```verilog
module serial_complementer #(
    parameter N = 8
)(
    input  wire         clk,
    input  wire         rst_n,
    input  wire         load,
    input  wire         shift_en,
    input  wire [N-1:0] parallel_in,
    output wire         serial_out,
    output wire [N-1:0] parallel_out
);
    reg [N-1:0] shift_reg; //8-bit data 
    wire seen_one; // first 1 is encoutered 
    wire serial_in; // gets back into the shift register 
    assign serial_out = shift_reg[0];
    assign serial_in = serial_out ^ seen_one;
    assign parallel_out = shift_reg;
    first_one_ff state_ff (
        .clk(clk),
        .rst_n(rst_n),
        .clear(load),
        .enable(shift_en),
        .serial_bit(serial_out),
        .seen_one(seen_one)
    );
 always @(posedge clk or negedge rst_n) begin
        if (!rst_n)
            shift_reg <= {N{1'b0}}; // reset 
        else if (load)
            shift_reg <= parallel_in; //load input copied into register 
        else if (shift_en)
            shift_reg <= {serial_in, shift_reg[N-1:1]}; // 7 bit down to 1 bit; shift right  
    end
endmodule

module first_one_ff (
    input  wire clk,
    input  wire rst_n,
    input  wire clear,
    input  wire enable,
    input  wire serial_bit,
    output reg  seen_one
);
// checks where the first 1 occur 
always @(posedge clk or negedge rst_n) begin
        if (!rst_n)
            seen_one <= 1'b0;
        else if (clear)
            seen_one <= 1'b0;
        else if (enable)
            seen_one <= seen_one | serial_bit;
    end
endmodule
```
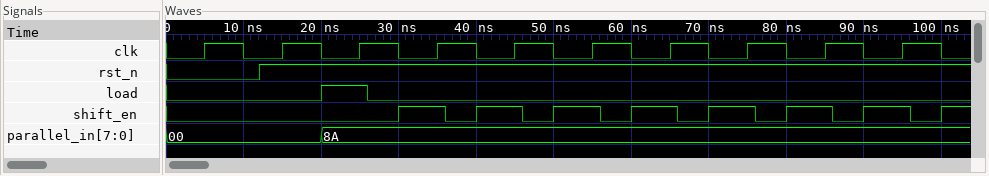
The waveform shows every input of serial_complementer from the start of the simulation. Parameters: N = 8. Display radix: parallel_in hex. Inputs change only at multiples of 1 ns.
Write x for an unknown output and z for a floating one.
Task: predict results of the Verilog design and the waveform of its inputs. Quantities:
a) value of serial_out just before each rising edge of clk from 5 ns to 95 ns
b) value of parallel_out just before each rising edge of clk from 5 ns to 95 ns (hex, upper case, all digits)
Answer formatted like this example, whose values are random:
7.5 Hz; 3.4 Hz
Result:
0 0 0 0 1 0 1 0 0 0; 00, 00, 00, 8A, 45, A2, D1, 68, B4, DA
